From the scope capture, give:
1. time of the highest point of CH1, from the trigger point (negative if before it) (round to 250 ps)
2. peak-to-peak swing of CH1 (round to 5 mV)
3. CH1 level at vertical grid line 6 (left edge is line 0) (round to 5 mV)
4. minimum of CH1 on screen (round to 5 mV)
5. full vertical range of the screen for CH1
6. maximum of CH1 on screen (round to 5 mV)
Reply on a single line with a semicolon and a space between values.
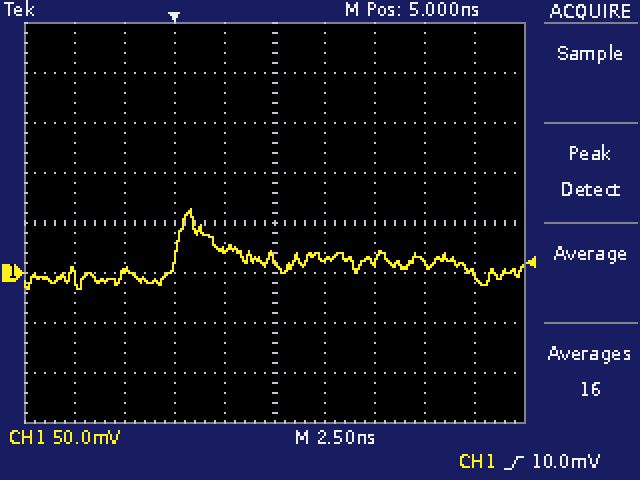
+750 ps; 80 mV; 15 mV; -15 mV; 400 mV; 65 mV
